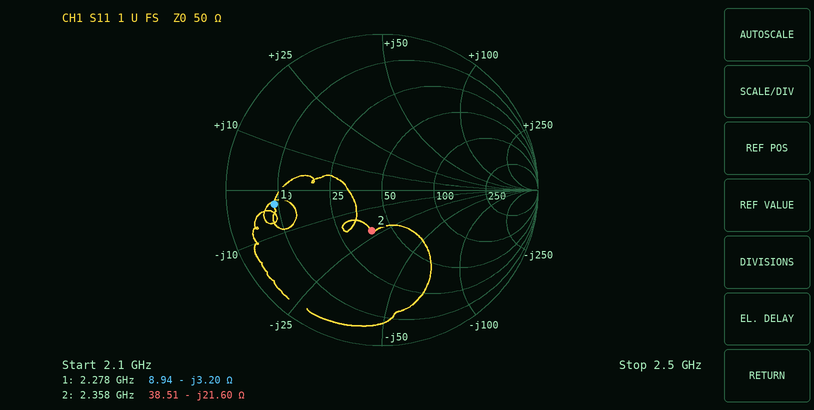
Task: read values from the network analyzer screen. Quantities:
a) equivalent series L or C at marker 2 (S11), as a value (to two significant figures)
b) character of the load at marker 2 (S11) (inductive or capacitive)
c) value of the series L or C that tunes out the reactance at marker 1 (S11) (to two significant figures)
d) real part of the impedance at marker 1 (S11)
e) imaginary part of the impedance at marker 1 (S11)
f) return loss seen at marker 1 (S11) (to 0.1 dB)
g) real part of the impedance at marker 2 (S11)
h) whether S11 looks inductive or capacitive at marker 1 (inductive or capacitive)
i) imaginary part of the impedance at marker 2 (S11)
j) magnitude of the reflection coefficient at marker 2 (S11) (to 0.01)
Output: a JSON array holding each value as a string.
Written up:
["3.1 pF", "capacitive", "220 pH", "8.94 Ω", "-3.20 Ω", "3.1 dB", "38.51 Ω", "capacitive", "-21.60 Ω", "0.27"]
